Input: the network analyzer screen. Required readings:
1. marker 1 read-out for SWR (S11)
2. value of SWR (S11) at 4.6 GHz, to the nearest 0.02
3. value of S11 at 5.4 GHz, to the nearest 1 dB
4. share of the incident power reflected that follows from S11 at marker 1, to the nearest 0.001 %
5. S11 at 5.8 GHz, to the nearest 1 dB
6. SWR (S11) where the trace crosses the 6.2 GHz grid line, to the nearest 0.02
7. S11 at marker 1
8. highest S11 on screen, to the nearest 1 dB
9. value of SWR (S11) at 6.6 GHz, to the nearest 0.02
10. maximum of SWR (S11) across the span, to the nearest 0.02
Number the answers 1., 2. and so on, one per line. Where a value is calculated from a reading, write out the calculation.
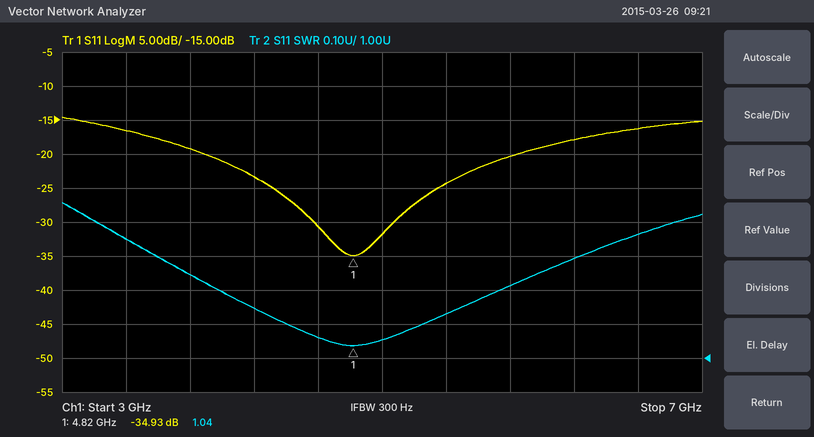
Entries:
1. 1.04
2. 1.06
3. -24 dB
4. 10^(-34.93/10) ≈ 0.032 %
5. -20 dB
6. 1.30
7. -34.93 dB
8. -15 dB
9. 1.36
10. 1.46
